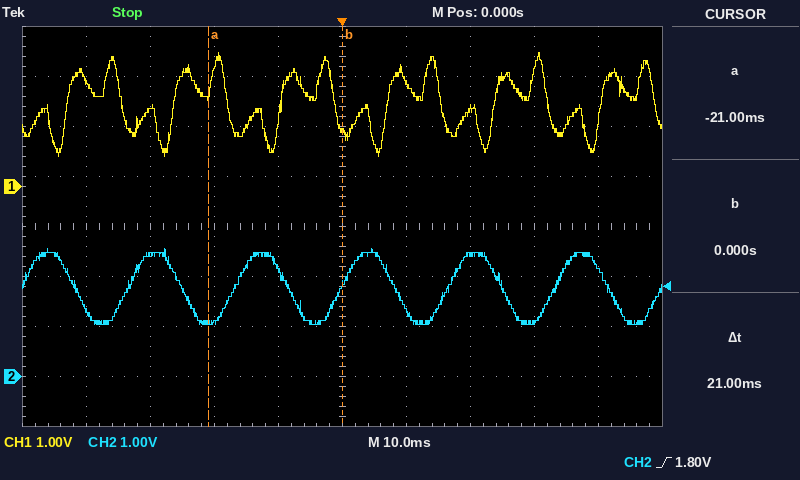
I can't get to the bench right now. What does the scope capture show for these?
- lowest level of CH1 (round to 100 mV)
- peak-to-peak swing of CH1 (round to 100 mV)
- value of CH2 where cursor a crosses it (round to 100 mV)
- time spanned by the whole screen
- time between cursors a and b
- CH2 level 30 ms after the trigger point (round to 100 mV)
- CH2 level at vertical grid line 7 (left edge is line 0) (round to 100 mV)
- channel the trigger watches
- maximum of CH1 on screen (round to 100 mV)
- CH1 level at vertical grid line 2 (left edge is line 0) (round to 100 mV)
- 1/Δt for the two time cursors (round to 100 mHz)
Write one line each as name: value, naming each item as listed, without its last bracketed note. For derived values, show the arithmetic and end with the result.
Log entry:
lowest level of CH1: 600 mV
peak-to-peak swing of CH1: 2.7 V − (600 mV) = 2.1 V
value of CH2 where cursor a crosses it: 1.1 V
time spanned by the whole screen: 100 ms
time between cursors a and b: 21 ms
CH2 level 30 ms after the trigger point: 1.1 V
CH2 level at vertical grid line 7 (left edge is line 0): 2.4 V
channel the trigger watches: CH2
maximum of CH1 on screen: 2.7 V
CH1 level at vertical grid line 2 (left edge is line 0): 1.6 V
1/Δt for the two time cursors: 1 / 21 ms ≈ 47.6 Hz
